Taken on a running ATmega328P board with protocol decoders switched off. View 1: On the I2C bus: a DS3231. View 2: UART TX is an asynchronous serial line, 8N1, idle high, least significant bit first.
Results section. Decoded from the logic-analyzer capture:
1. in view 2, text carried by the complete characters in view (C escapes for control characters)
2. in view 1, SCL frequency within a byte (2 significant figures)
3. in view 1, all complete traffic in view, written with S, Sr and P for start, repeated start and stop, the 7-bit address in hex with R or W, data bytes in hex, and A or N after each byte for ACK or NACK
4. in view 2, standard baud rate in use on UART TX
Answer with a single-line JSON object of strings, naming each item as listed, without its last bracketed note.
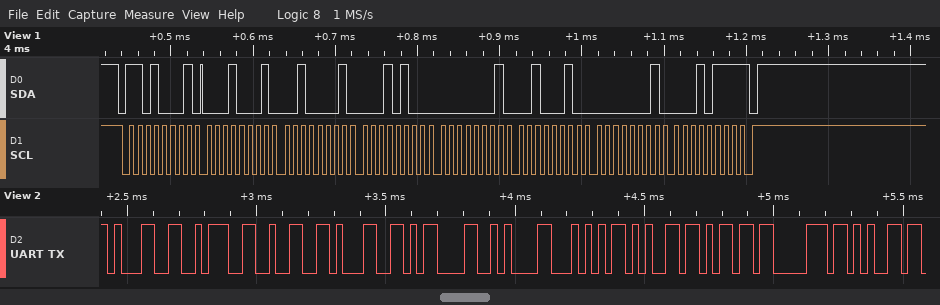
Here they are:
{"in view 2, text carried by the complete characters in view": "\"1:21\\r\\nTempe\"", "in view 1, SCL frequency within a byte": "100 kHz", "in view 1, all complete traffic in view, written with S, Sr and P for start, repeated start and stop, the 7-bit address in hex with R or W, data bytes in hex, and A or N after each byte for ACK or NACK": "S 68R A 11 A 21 A 14 A 01 A 22 A 01 A 17 N P", "in view 2, standard baud rate in use on UART TX": "38400 baud"}
